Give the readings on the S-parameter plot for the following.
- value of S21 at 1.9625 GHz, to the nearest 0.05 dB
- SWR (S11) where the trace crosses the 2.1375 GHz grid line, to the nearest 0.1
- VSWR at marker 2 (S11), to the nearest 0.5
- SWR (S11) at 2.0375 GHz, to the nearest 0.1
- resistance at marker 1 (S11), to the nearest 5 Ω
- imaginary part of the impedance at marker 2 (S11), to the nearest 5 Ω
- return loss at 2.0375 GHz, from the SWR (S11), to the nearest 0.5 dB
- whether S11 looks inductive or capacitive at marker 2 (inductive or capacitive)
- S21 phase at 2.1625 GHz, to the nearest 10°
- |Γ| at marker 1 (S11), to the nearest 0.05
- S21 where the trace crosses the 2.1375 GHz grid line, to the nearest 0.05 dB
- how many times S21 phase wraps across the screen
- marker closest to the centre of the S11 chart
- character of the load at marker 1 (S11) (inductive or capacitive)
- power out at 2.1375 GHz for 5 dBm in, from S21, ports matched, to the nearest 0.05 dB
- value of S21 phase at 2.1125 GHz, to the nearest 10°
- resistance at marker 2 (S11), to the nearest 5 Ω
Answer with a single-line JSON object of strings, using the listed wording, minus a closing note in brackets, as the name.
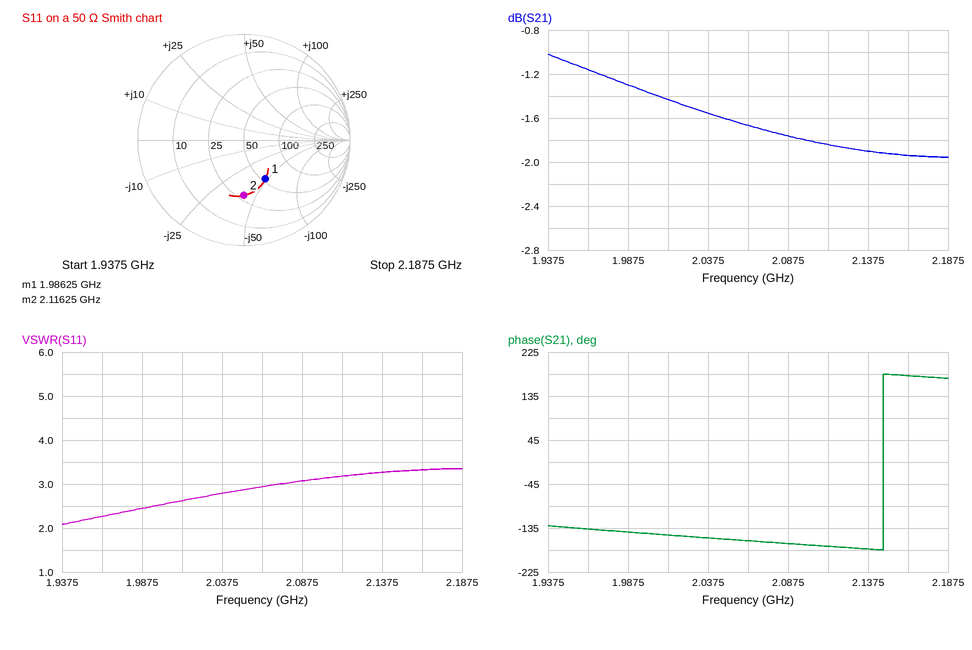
{"value of S21 at 1.9625 GHz, to the nearest 0.05 dB": "-1.15 dB", "SWR (S11) where the trace crosses the 2.1375 GHz grid line, to the nearest 0.1": "3.3", "VSWR at marker 2 (S11), to the nearest 0.5": "3.0", "SWR (S11) at 2.0375 GHz, to the nearest 0.1": "2.8", "resistance at marker 1 (S11), to the nearest 5 Ω": "55 Ω", "imaginary part of the impedance at marker 2 (S11), to the nearest 5 Ω": "-40 Ω", "return loss at 2.0375 GHz, from the SWR (S11), to the nearest 0.5 dB": "6.5 dB", "whether S11 looks inductive or capacitive at marker 2": "capacitive", "S21 phase at 2.1625 GHz, to the nearest 10°": "180°", "|Γ| at marker 1 (S11), to the nearest 0.05": "0.40", "S21 where the trace crosses the 2.1375 GHz grid line, to the nearest 0.05 dB": "-1.90 dB", "how many times S21 phase wraps across the screen": "1", "marker closest to the centre of the S11 chart": "marker 1", "character of the load at marker 1 (S11)": "capacitive", "power out at 2.1375 GHz for 5 dBm in, from S21, ports matched, to the nearest 0.05 dB": "3.10 dBm", "value of S21 phase at 2.1125 GHz, to the nearest 10°": "-170°", "resistance at marker 2 (S11), to the nearest 5 Ω": "30 Ω"}
